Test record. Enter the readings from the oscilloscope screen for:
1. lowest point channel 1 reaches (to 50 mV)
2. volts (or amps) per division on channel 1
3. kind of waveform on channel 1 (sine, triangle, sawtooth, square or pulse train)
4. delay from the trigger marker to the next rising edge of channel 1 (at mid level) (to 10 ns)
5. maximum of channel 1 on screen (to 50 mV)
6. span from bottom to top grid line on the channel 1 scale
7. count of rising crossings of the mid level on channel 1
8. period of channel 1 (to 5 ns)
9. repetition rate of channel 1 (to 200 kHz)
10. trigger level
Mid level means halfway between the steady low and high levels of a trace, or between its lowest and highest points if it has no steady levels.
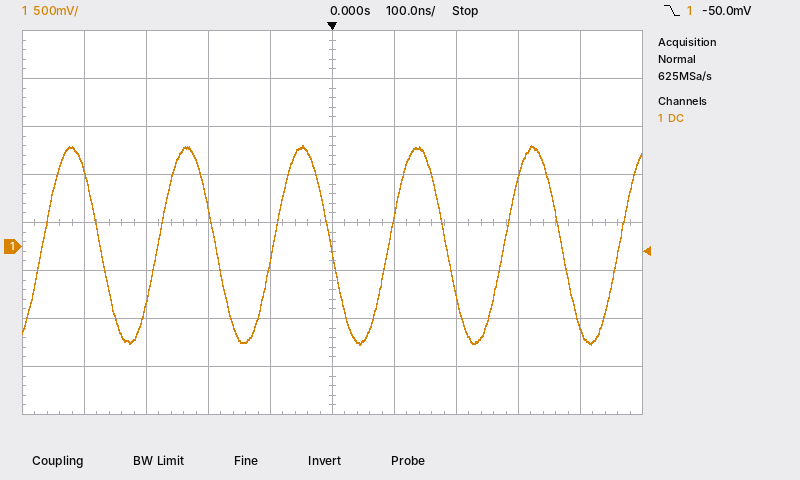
-1.00 V
500 mV
sine
90 ns
1.05 V
4 V
6
185 ns
5.4 MHz
-50.0 mV
